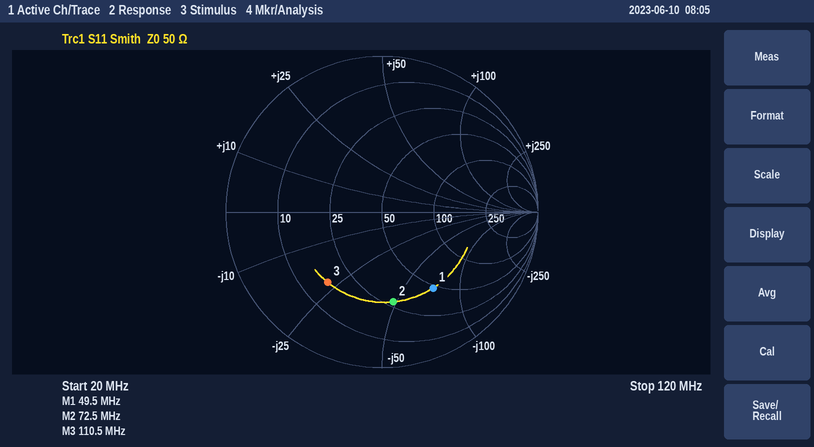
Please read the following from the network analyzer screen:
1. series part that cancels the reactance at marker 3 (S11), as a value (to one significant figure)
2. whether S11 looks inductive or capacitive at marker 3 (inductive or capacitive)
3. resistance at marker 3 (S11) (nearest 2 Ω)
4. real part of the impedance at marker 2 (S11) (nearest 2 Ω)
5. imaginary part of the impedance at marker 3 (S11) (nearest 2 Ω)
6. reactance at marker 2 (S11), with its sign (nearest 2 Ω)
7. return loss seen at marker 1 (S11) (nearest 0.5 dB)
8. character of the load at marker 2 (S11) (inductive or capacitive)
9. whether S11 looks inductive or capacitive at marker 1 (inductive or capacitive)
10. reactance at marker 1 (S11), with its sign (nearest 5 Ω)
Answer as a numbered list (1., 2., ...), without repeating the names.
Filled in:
1. 30 nH
2. capacitive
3. 16 Ω
4. 28 Ω
5. -22 Ω
6. -48 Ω
7. 4.5 dB
8. capacitive
9. capacitive
10. -70 Ω
